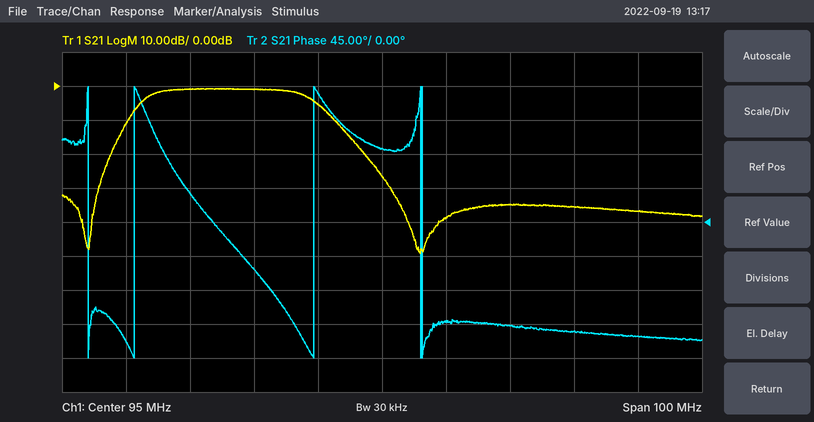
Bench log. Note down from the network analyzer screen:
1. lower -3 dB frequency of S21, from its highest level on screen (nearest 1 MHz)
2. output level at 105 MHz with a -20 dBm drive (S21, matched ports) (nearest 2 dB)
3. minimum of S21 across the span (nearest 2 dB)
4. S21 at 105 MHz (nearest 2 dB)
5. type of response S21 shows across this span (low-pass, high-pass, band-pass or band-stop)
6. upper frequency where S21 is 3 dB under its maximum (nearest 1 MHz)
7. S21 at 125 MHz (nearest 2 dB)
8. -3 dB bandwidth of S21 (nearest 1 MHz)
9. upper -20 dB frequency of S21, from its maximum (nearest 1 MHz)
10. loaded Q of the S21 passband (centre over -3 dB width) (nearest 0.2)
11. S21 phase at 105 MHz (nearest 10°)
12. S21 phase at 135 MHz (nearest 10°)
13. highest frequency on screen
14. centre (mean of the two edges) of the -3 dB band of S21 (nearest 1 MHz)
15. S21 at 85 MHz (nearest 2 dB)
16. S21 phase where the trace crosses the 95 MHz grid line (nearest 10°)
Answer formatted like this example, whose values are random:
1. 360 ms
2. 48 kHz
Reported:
1. 58 MHz
2. -58 dBm
3. -50 dB
4. -38 dB
5. band-pass
6. 84 MHz
7. -36 dB
8. 26 MHz
9. 93 MHz
10. 2.8
11. -130°
12. -150°
13. 145 MHz
14. 71 MHz
15. -6 dB
16. 100°
